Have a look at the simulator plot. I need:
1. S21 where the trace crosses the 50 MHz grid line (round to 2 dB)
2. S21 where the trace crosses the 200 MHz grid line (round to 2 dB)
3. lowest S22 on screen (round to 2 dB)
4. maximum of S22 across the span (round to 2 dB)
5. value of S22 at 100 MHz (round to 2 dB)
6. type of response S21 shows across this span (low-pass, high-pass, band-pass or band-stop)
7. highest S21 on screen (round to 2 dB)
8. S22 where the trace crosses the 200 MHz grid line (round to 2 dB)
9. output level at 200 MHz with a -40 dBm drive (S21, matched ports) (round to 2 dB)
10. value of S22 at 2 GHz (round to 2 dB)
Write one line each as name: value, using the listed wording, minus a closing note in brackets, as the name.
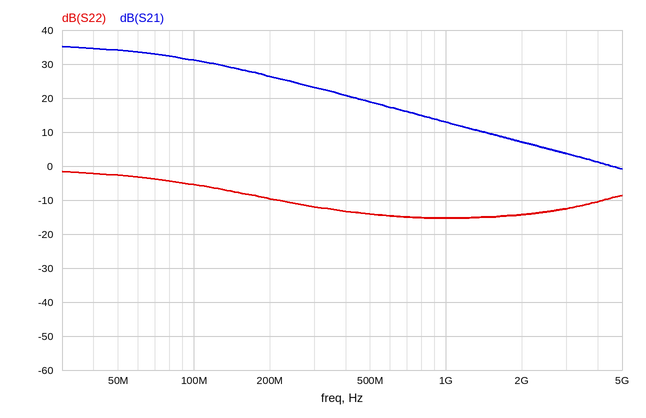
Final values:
S21 where the trace crosses the 50 MHz grid line: 34 dB
S21 where the trace crosses the 200 MHz grid line: 26 dB
lowest S22 on screen: -16 dB
maximum of S22 across the span: -2 dB
value of S22 at 100 MHz: -6 dB
type of response S21 shows across this span: low-pass
highest S21 on screen: 36 dB
S22 where the trace crosses the 200 MHz grid line: -10 dB
output level at 200 MHz with a -40 dBm drive (S21, matched ports): -14 dBm
value of S22 at 2 GHz: -14 dB
